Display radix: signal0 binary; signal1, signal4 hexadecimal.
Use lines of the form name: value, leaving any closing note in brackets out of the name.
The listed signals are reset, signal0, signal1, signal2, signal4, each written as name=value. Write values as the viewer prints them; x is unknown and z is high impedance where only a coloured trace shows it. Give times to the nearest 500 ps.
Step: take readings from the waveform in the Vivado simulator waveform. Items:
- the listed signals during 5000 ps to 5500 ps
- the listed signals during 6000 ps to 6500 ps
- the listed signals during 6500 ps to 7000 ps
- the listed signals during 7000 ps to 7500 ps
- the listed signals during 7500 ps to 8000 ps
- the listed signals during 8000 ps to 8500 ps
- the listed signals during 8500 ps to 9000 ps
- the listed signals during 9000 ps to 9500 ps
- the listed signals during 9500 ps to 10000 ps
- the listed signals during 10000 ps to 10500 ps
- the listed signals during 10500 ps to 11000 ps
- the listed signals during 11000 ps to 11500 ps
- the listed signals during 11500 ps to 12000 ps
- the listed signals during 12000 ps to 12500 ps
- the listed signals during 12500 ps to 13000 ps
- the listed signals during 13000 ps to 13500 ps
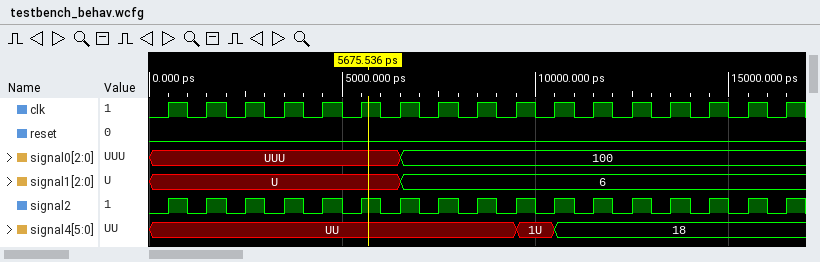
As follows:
the listed signals during 5000 ps to 5500 ps: reset=0, signal0=UUU, signal1=U, signal2=0, signal4=UU
the listed signals during 6000 ps to 6500 ps: reset=0, signal0=UUU, signal1=U, signal2=0, signal4=UU
the listed signals during 6500 ps to 7000 ps: reset=0, signal0=100, signal1=6, signal2=1, signal4=UU
the listed signals during 7000 ps to 7500 ps: reset=0, signal0=100, signal1=6, signal2=0, signal4=UU
the listed signals during 7500 ps to 8000 ps: reset=0, signal0=100, signal1=6, signal2=1, signal4=UU
the listed signals during 8000 ps to 8500 ps: reset=0, signal0=100, signal1=6, signal2=0, signal4=UU
the listed signals during 8500 ps to 9000 ps: reset=0, signal0=100, signal1=6, signal2=1, signal4=UU
the listed signals during 9000 ps to 9500 ps: reset=0, signal0=100, signal1=6, signal2=0, signal4=UU
the listed signals during 9500 ps to 10000 ps: reset=0, signal0=100, signal1=6, signal2=1, signal4=1U
the listed signals during 10000 ps to 10500 ps: reset=0, signal0=100, signal1=6, signal2=0, signal4=1U
the listed signals during 10500 ps to 11000 ps: reset=0, signal0=100, signal1=6, signal2=1, signal4=18
the listed signals during 11000 ps to 11500 ps: reset=0, signal0=100, signal1=6, signal2=0, signal4=18
the listed signals during 11500 ps to 12000 ps: reset=0, signal0=100, signal1=6, signal2=1, signal4=18
the listed signals during 12000 ps to 12500 ps: reset=0, signal0=100, signal1=6, signal2=0, signal4=18
the listed signals during 12500 ps to 13000 ps: reset=0, signal0=100, signal1=6, signal2=1, signal4=18
the listed signals during 13000 ps to 13500 ps: reset=0, signal0=100, signal1=6, signal2=0, signal4=18
